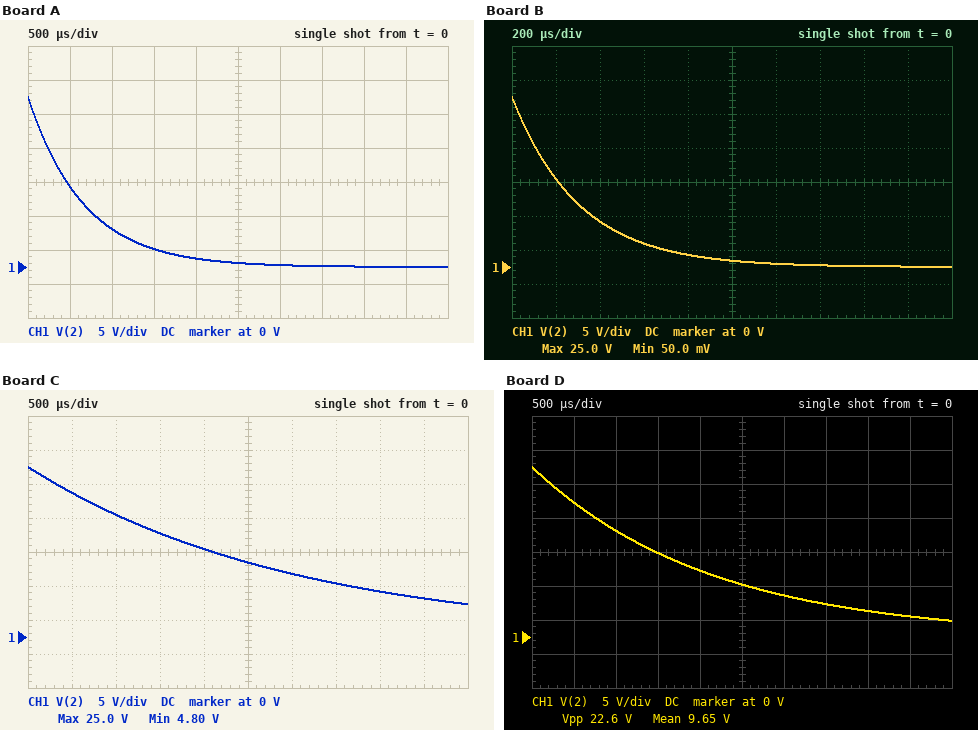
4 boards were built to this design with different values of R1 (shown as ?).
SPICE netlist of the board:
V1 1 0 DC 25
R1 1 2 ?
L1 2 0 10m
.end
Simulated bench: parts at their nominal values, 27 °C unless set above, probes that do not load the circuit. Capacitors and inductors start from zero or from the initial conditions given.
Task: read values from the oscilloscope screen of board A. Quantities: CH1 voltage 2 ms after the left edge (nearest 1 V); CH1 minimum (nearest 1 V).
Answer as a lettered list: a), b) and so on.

a) 1 V
b) 0 V
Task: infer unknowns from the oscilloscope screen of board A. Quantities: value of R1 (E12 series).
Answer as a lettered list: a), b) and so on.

a) 15 Ω
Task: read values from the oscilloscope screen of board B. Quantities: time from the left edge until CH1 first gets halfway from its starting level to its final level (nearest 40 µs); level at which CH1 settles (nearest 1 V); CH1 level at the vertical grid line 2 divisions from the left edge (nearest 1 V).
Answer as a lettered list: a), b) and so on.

a) 200 µs
b) 0 V
c) 7 V
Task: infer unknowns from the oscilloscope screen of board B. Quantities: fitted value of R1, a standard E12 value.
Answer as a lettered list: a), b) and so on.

a) 33 Ω
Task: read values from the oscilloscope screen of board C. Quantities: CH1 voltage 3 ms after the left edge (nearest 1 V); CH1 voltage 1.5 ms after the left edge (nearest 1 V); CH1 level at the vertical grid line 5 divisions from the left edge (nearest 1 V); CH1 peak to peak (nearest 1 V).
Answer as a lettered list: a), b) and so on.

a) 9 V
b) 15 V
c) 11 V
d) 20 V
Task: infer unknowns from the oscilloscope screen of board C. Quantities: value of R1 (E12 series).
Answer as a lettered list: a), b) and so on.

a) 3.3 Ω
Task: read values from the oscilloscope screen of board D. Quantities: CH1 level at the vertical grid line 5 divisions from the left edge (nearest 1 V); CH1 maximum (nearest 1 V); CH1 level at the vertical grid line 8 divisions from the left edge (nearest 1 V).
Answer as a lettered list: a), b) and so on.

a) 8 V
b) 25 V
c) 4 V
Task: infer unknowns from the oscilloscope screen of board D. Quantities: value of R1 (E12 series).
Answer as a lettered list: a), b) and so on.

a) 4.7 Ω
